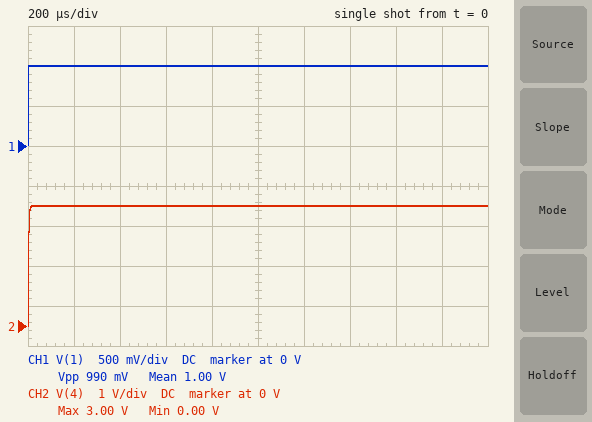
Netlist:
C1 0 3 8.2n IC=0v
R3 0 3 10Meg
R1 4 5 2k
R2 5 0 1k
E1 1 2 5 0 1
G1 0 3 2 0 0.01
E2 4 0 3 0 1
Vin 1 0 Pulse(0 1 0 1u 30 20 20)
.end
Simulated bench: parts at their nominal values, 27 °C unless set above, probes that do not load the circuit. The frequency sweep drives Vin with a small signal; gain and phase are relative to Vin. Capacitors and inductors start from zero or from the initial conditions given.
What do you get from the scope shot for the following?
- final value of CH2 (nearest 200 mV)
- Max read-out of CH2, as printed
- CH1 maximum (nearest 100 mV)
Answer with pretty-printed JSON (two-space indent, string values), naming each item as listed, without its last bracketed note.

{
  "final value of CH2": "3.0 V",
  "Max read-out of CH2, as printed": "3.00 V",
  "CH1 maximum": "1.0 V"
}
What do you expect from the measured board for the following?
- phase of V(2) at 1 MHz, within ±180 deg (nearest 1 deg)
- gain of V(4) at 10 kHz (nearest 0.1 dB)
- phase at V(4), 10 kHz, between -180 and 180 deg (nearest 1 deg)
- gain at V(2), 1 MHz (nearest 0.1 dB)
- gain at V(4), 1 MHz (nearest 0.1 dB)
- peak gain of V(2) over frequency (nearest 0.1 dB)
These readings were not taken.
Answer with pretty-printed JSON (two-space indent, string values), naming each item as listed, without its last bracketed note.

{
  "phase of V(2) at 1 MHz, within ±180 deg": "4 deg",
  "gain of V(4) at 10 kHz": "9.4 dB",
  "phase at V(4), 10 kHz, between -180 and 180 deg": "-9 deg",
  "gain at V(2), 1 MHz": "0 dB",
  "gain at V(4), 1 MHz": "-14.3 dB",
  "peak gain of V(2) over frequency": "0 dB"
}
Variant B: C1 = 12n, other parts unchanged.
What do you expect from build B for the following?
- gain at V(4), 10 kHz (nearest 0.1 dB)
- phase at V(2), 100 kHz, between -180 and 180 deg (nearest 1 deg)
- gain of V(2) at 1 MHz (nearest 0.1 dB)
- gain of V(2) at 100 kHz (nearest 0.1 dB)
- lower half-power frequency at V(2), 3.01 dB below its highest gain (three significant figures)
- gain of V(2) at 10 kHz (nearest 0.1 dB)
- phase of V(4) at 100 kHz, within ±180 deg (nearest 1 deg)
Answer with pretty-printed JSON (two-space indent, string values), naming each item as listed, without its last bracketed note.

{
  "gain at V(4), 10 kHz": "9.3 dB",
  "phase at V(2), 100 kHz, between -180 and 180 deg": "24 deg",
  "gain of V(2) at 1 MHz": "0 dB",
  "gain of V(2) at 100 kHz": "-0.8 dB",
  "lower half-power frequency at V(2), 3.01 dB below its highest gain": "44.2 kHz",
  "gain of V(2) at 10 kHz": "-13.1 dB",
  "phase of V(4) at 100 kHz, within ±180 deg": "-66 deg"
}
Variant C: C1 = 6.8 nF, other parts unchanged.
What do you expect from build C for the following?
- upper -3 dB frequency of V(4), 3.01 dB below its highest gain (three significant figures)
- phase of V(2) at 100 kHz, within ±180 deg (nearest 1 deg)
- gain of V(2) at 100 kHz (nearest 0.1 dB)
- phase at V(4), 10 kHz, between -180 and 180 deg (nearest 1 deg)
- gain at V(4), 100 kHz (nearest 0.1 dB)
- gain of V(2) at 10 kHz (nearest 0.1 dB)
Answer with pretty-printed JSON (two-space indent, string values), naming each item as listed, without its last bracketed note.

{
  "upper -3 dB frequency of V(4), 3.01 dB below its highest gain": "78.0 kHz",
  "phase of V(2) at 100 kHz, within ±180 deg": "38 deg",
  "gain of V(2) at 100 kHz": "-2.1 dB",
  "phase at V(4), 10 kHz, between -180 and 180 deg": "-7 deg",
  "gain at V(4), 100 kHz": "5.3 dB",
  "gain of V(2) at 10 kHz": "-17.9 dB"
}
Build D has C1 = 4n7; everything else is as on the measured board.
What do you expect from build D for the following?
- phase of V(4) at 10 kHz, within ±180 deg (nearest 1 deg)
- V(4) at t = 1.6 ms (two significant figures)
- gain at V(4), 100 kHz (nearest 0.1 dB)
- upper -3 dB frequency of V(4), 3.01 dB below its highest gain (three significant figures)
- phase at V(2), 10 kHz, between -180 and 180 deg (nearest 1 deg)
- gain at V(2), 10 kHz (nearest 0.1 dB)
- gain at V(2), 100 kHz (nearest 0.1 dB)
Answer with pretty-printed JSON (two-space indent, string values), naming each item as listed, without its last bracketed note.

{
  "phase of V(4) at 10 kHz, within ±180 deg": "-5 deg",
  "V(4) at t = 1.6 ms": "3.0 V",
  "gain at V(4), 100 kHz": "7.0 dB",
  "upper -3 dB frequency of V(4), 3.01 dB below its highest gain": "113 kHz",
  "phase at V(2), 10 kHz, between -180 and 180 deg": "85 deg",
  "gain at V(2), 10 kHz": "-21.1 dB",
  "gain at V(2), 100 kHz": "-3.6 dB"
}
